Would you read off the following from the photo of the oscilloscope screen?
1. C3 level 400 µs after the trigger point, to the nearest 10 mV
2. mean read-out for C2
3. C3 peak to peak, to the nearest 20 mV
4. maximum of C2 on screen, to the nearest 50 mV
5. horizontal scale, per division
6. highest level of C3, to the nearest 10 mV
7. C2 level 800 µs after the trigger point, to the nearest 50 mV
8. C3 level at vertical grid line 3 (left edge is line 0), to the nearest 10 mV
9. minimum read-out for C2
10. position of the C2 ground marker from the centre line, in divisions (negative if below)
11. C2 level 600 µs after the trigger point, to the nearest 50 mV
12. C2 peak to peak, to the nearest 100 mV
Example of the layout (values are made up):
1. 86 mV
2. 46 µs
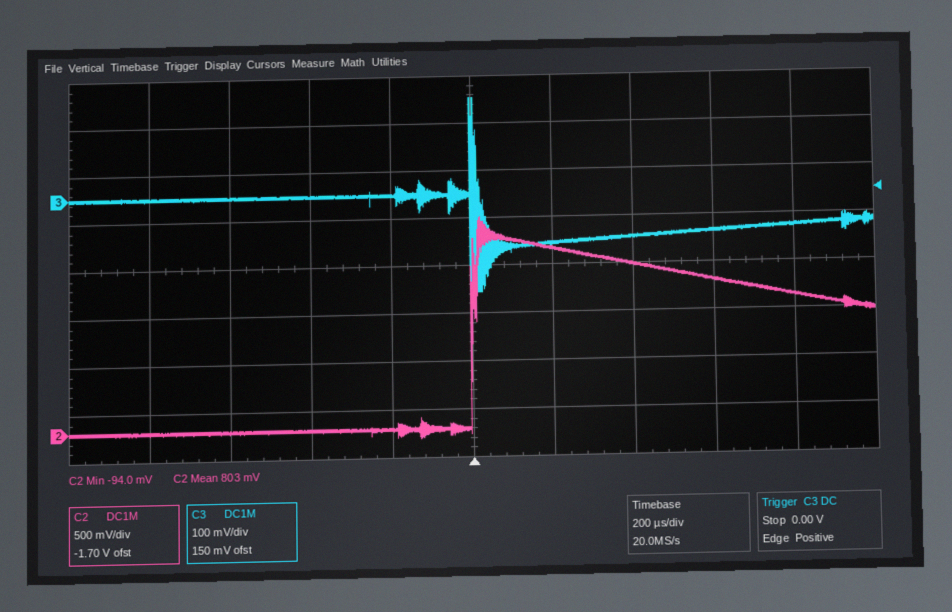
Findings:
1. -90 mV
2. 803 mV
3. 400 mV
4. 2.20 V
5. 200 µs
6. 200 mV
7. 1.35 V
8. 0 mV
9. -94.0 mV
10. -3.4 div
11. 1.50 V
12. 2.30 V
